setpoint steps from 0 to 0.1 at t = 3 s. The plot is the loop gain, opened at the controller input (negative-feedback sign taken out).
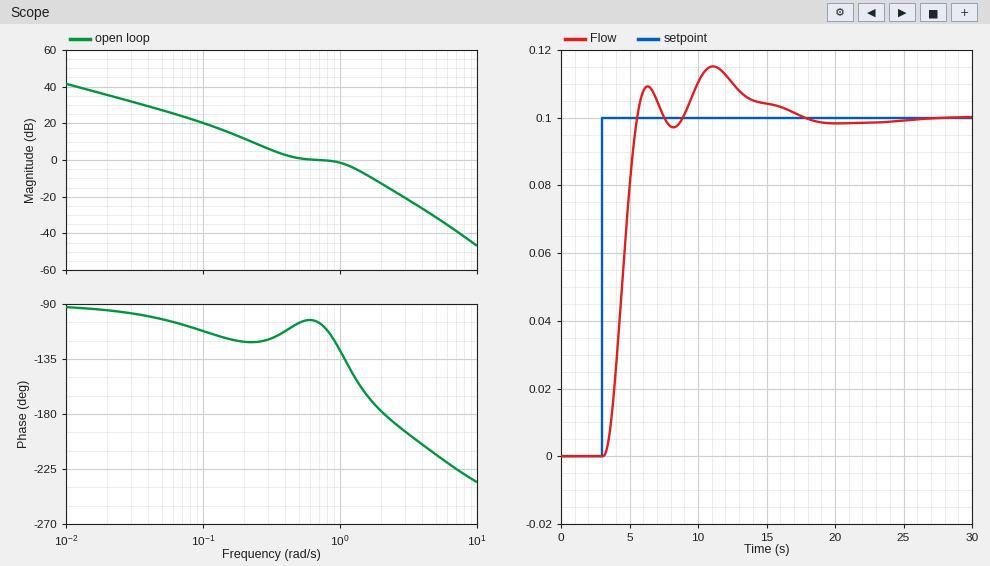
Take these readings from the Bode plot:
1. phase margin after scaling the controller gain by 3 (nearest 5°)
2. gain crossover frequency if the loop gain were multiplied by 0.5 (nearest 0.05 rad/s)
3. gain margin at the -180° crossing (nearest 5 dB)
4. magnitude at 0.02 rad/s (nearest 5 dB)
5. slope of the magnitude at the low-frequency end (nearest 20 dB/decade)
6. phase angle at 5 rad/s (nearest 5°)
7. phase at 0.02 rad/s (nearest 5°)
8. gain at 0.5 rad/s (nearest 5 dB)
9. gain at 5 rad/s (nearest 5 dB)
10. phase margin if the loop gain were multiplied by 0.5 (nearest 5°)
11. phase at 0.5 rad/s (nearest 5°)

10°
0.30 rad/s
15 dB
35 dB
-20 dB/decade
-215°
-95°
0 dB
-30 dB
60°
-105°
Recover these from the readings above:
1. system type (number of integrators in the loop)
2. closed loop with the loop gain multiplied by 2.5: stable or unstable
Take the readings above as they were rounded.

1
stable
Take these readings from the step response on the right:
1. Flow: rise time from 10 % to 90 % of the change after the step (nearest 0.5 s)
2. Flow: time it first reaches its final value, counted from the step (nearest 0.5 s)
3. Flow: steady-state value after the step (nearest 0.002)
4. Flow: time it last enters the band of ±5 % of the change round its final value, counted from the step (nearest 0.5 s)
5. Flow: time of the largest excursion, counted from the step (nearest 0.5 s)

1.5 s
2.5 s
0.100
11.0 s
8.0 s
